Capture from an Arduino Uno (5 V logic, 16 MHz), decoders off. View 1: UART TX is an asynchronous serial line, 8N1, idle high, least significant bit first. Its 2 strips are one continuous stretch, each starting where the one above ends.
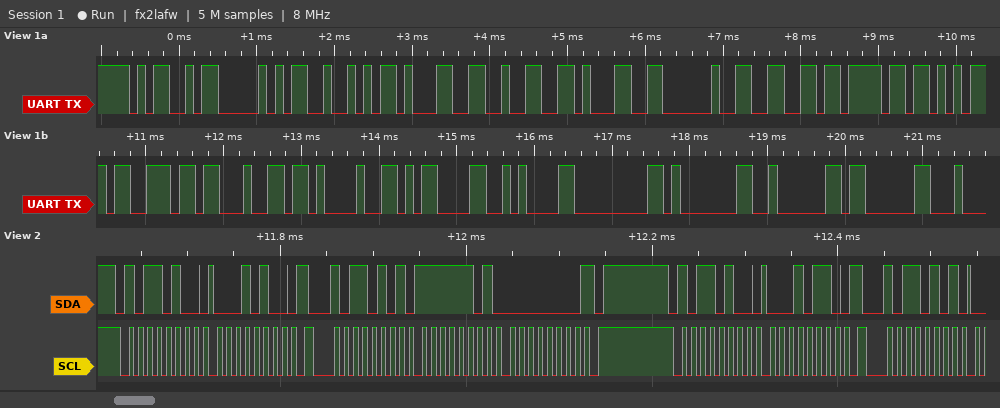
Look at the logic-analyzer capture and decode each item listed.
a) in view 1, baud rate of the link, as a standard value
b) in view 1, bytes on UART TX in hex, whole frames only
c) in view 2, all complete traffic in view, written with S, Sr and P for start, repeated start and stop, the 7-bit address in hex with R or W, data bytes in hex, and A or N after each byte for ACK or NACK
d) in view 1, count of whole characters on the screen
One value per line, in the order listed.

9600 baud
4D 50 52 31 32 31 20 66 6F 75 6E 64 21 0D 0A 00 01 02 03
S 5AW A 14 A Sr 5AR A FD A 00 N P S 5AW A 16 A Sr 5AR A
19
